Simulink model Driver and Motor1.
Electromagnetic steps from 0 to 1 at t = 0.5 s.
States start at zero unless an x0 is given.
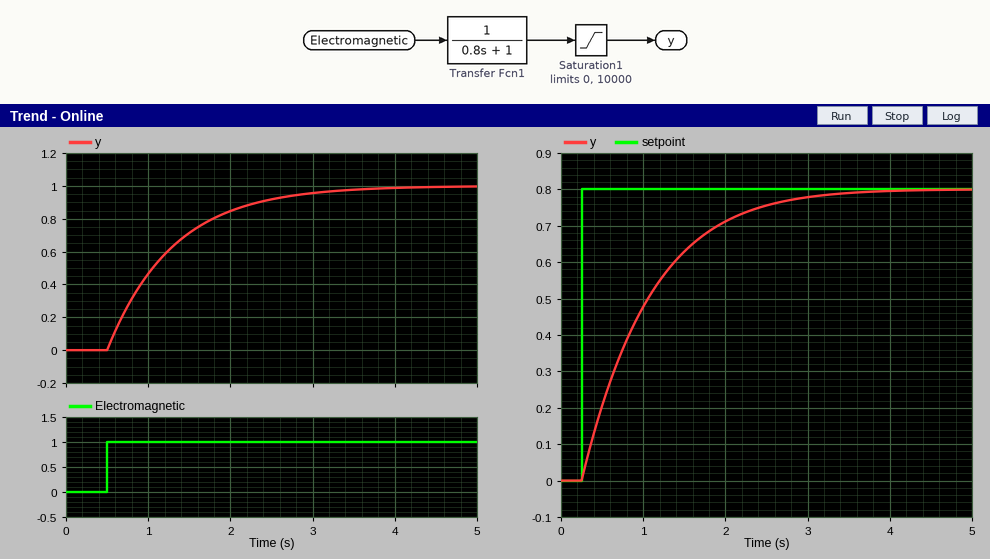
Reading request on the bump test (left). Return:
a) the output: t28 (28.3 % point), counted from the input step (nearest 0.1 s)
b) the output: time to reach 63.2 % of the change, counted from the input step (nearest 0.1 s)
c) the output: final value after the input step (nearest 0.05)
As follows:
0.3 s
0.8 s
1.00
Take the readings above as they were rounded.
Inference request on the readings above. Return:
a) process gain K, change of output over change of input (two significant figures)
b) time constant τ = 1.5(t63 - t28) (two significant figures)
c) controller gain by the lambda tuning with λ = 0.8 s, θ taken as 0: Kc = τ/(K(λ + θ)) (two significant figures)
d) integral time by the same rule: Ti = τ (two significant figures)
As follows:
1.0
0.75 s
0.94
0.75 s
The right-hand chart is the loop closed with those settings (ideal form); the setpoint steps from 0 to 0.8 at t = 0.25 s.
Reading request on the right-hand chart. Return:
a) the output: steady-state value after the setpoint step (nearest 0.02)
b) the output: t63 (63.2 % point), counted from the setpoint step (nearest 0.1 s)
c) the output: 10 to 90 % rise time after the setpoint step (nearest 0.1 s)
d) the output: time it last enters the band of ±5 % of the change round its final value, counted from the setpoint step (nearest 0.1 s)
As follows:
0.80
0.8 s
1.7 s
2.3 s
